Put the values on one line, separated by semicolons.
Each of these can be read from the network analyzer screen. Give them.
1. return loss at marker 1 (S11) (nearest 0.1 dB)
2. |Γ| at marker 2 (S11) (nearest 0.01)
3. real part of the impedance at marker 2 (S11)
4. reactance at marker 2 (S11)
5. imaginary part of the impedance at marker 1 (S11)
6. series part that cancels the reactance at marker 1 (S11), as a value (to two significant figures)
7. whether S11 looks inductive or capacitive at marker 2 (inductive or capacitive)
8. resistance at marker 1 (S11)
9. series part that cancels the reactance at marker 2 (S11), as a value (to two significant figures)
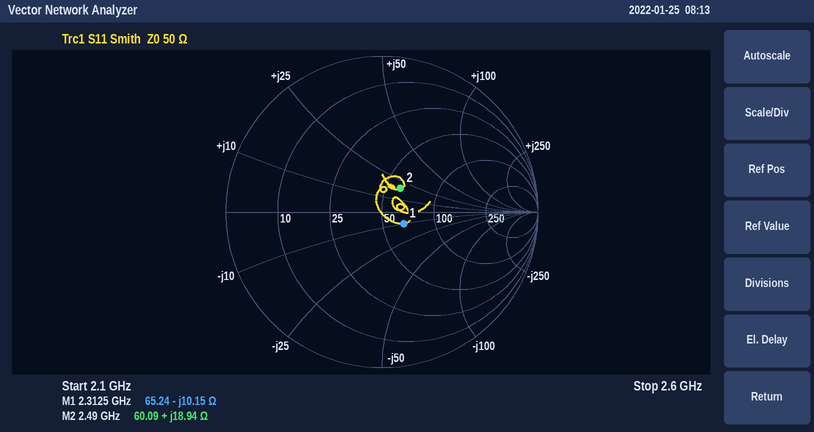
16.0 dB; 0.19; 60.09 Ω; +18.94 Ω; -10.15 Ω; 700 pH; inductive; 65.24 Ω; 3.4 pF
